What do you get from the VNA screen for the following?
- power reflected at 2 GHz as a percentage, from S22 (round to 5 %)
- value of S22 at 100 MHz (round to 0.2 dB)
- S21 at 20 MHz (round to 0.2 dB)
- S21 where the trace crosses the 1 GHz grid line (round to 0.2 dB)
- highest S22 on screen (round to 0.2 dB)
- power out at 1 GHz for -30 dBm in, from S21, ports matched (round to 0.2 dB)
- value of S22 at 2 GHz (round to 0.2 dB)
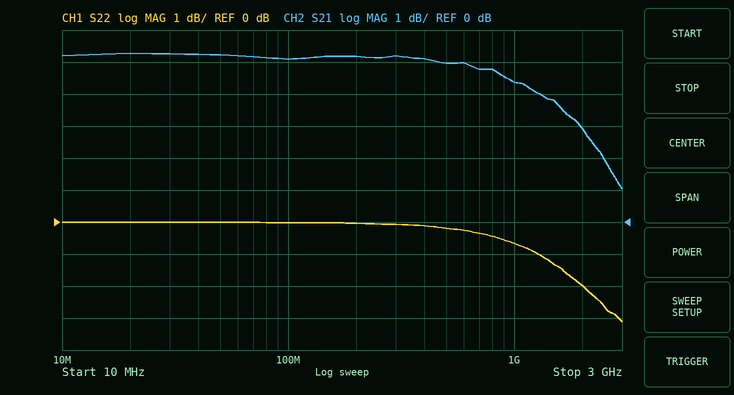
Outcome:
65 %
0.0 dB
5.2 dB
4.4 dB
0.0 dB
-25.6 dBm
-2.0 dB
